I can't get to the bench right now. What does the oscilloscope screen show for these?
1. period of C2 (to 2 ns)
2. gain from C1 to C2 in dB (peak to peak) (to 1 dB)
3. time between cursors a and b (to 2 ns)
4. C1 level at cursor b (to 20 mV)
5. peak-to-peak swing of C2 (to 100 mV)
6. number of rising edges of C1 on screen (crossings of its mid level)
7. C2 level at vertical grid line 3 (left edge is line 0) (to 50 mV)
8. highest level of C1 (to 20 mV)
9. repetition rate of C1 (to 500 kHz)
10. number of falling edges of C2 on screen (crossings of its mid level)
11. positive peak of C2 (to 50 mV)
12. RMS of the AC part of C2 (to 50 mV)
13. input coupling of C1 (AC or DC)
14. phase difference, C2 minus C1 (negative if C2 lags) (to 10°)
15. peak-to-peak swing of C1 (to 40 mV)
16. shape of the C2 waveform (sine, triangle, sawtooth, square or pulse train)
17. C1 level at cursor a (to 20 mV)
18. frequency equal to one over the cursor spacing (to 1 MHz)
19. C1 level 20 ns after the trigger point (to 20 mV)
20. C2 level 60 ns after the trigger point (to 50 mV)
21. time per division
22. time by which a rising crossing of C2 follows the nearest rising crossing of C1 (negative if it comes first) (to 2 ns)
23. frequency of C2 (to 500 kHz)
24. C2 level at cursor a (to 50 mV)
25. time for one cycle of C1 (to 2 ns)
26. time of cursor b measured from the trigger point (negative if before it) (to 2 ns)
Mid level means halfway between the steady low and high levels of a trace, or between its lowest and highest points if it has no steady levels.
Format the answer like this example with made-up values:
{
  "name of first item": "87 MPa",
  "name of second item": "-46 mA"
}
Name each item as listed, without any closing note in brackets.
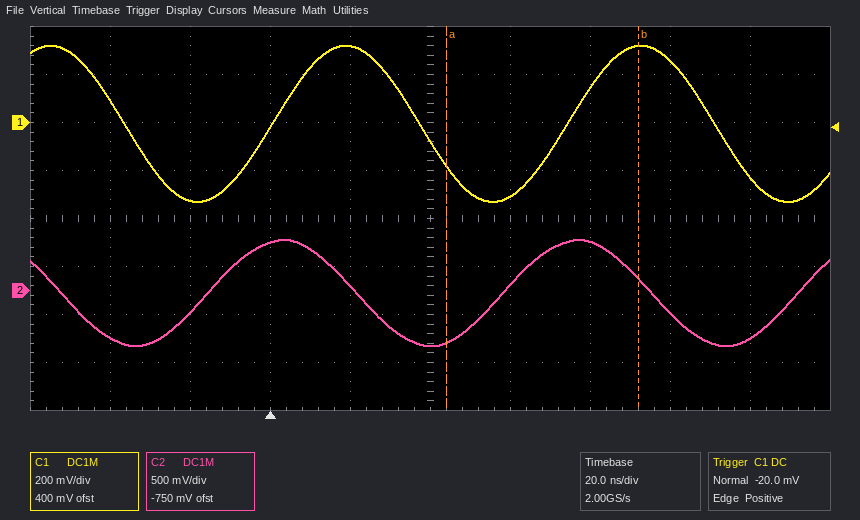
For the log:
{
  "period of C2": "74 ns",
  "gain from C1 to C2 in dB (peak to peak)": "5 dB",
  "time between cursors a and b": "48 ns",
  "C1 level at cursor b": "320 mV",
  "peak-to-peak swing of C2": "1.10 V",
  "number of rising edges of C1 on screen": "2",
  "C2 level at vertical grid line 3 (left edge is line 0)": "500 mV",
  "highest level of C1": "320 mV",
  "repetition rate of C1": "13.5 MHz",
  "number of falling edges of C2 on screen": "3",
  "positive peak of C2": "550 mV",
  "RMS of the AC part of C2": "400 mV",
  "input coupling of C1": "DC",
  "phase difference, C2 minus C1 (negative if C2 lags)": "+80°",
  "peak-to-peak swing of C1": "640 mV",
  "shape of the C2 waveform": "sine",
  "C1 level at cursor a": "-180 mV",
  "frequency equal to one over the cursor spacing": "21 MHz",
  "C1 level 20 ns after the trigger point": "320 mV",
  "C2 level 60 ns after the trigger point": "50 mV",
  "time per division": "20 ns",
  "time by which a rising crossing of C2 follows the nearest rising crossing of C1 (negative if it comes first)": "-16 ns",
  "frequency of C2": "13.5 MHz",
  "C2 level at cursor a": "-550 mV",
  "time for one cycle of C1": "74 ns",
  "time of cursor b measured from the trigger point (negative if before it)": "+92 ns"
}
